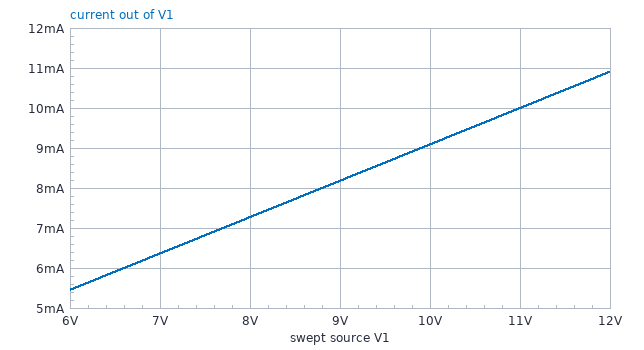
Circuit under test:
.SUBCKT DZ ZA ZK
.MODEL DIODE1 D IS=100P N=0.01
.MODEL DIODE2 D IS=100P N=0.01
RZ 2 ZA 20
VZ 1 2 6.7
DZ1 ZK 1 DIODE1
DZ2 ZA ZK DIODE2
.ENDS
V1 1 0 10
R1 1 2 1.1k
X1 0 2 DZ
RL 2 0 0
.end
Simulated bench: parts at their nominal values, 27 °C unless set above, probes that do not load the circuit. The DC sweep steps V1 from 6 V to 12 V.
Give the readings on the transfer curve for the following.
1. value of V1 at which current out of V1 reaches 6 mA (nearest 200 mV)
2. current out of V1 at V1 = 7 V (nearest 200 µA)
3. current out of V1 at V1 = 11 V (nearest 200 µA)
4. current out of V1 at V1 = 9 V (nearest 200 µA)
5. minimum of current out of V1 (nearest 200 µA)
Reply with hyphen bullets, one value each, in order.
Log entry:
- 6.6 V
- 6.4 mA
- 10.0 mA
- 8.2 mA
- 5.4 mA
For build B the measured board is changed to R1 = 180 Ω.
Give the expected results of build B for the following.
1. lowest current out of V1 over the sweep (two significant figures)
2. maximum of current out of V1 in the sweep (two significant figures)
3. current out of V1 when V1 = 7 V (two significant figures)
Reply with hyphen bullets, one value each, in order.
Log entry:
- 33 mA
- 67 mA
- 39 mA
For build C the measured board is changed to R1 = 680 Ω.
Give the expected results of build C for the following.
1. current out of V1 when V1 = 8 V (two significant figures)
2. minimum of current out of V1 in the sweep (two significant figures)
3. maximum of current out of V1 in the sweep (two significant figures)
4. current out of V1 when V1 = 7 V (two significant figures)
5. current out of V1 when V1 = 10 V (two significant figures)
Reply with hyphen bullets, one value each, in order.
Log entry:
- 12 mA
- 8.8 mA
- 18 mA
- 10 mA
- 15 mA
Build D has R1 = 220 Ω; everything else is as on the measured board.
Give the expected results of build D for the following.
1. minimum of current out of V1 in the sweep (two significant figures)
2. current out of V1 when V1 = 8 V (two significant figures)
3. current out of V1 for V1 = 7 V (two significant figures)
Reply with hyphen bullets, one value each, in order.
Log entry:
- 27 mA
- 36 mA
- 32 mA
